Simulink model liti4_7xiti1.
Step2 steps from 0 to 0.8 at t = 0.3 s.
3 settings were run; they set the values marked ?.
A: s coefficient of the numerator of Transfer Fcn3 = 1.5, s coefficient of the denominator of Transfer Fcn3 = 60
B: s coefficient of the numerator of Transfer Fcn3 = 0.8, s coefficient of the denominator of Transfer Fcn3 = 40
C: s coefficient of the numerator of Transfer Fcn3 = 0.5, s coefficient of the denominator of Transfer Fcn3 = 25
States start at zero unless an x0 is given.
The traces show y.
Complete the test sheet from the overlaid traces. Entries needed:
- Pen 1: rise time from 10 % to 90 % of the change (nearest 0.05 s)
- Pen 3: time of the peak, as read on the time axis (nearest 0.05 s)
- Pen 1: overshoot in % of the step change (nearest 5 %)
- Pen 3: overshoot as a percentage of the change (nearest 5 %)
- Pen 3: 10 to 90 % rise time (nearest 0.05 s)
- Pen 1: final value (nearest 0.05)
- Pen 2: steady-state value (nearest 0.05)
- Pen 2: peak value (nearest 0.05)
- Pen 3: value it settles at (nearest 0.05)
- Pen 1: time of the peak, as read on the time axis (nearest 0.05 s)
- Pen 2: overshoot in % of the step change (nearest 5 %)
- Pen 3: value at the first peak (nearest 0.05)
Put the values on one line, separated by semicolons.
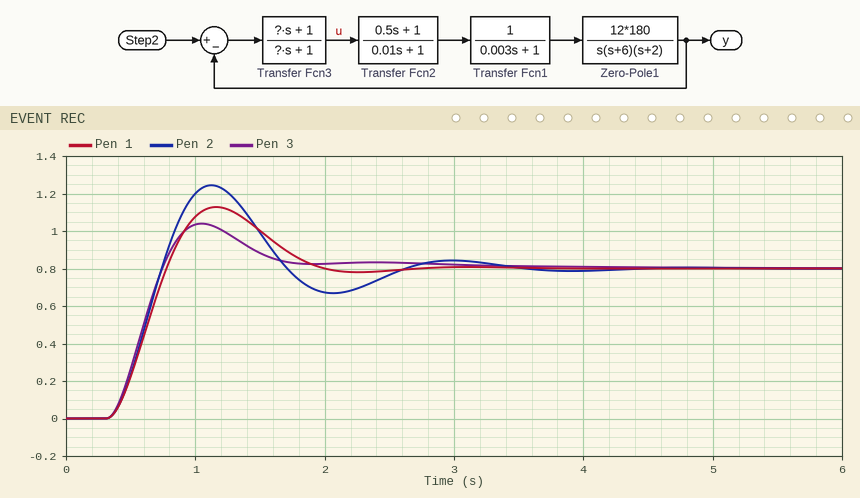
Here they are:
0.30 s; 1.05 s; 40 %; 30 %; 0.30 s; 0.80; 0.80; 1.25; 0.80; 1.15 s; 55 %; 1.05
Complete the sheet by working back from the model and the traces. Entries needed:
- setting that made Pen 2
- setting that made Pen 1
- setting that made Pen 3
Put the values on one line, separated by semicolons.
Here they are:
C; B; A
